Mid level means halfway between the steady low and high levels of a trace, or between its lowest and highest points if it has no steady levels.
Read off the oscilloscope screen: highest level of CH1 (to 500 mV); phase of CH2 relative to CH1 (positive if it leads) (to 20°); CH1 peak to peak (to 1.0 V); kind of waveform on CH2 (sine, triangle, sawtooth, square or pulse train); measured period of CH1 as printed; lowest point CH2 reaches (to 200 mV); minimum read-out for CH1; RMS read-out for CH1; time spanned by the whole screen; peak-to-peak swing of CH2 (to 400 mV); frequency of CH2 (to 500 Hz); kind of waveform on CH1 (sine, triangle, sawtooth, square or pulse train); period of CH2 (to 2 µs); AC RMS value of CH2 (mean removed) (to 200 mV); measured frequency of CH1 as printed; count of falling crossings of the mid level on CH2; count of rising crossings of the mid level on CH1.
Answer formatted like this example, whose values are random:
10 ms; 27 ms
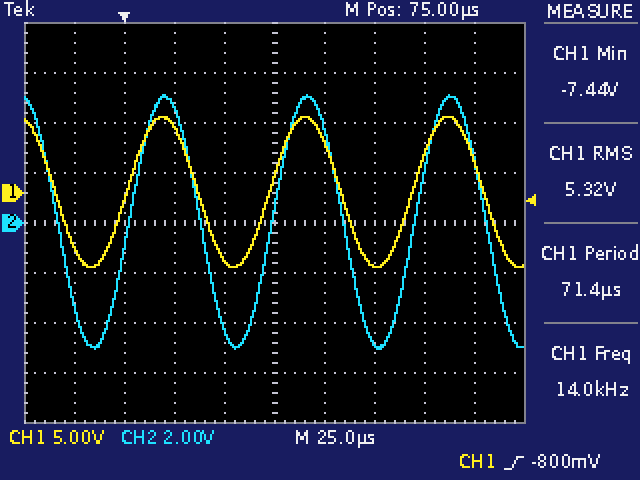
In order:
7.5 V; 0°; 15.0 V; sine; 71.4 µs; -5.0 V; -7.44 V; 5.32 V; 250 µs; 10.0 V; 14.0 kHz; sine; 72 µs; 3.6 V; 14.0 kHz; 4; 3
